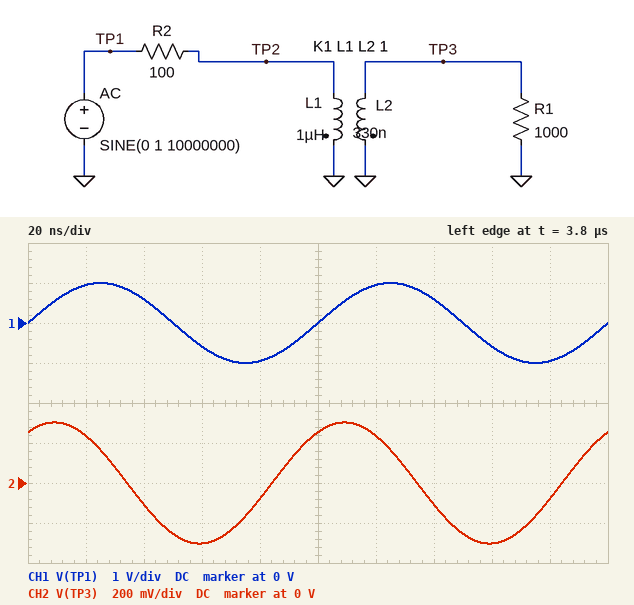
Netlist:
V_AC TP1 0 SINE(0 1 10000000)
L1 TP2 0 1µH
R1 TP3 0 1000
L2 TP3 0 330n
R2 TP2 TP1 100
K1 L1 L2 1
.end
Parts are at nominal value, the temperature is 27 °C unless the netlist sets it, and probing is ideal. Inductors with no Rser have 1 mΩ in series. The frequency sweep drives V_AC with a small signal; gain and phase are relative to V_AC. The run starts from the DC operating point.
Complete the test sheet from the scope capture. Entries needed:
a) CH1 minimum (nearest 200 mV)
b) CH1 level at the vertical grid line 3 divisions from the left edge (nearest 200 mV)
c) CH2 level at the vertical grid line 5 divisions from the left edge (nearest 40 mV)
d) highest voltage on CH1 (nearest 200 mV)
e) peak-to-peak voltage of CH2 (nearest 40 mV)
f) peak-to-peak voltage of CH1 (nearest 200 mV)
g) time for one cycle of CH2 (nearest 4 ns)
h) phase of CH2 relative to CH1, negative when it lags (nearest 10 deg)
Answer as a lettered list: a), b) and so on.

a) -1.0 V
b) -600 mV
c) 240 mV
d) 1.0 V
e) 600 mV
f) 2.0 V
g) 100 ns
h) 60 deg
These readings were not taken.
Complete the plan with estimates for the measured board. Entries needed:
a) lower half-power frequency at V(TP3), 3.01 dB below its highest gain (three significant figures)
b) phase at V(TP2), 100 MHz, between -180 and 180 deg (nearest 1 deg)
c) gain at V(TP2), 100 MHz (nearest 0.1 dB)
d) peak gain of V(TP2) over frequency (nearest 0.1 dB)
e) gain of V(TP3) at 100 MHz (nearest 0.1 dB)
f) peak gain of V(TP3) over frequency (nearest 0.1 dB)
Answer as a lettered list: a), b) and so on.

a) 15.4 MHz
b) 9 deg
c) -0.4 dB
d) -0.3 dB
e) -5.2 dB
f) -5.1 dB
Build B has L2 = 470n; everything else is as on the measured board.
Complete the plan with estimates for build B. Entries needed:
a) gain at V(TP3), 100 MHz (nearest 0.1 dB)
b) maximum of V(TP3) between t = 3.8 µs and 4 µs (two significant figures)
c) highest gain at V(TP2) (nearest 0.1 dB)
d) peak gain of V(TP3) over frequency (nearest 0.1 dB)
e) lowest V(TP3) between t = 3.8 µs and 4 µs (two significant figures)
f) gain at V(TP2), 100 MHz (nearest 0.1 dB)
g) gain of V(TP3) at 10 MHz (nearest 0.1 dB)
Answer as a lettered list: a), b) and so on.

a) -3.8 dB
b) 360 mV
c) -0.4 dB
d) -3.7 dB
e) -360 mV
f) -0.5 dB
g) -8.9 dB
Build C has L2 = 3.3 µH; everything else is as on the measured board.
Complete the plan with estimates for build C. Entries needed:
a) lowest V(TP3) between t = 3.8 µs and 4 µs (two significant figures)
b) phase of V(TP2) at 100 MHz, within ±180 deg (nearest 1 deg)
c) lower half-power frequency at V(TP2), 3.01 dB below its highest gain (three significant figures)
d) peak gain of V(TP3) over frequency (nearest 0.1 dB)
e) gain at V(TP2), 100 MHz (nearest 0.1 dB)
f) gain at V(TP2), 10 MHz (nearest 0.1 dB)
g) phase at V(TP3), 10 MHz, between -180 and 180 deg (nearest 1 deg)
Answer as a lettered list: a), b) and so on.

a) -880 mV
b) 7 deg
c) 12.0 MHz
d) 2.7 dB
e) -2.5 dB
f) -6.3 dB
g) 50 deg
